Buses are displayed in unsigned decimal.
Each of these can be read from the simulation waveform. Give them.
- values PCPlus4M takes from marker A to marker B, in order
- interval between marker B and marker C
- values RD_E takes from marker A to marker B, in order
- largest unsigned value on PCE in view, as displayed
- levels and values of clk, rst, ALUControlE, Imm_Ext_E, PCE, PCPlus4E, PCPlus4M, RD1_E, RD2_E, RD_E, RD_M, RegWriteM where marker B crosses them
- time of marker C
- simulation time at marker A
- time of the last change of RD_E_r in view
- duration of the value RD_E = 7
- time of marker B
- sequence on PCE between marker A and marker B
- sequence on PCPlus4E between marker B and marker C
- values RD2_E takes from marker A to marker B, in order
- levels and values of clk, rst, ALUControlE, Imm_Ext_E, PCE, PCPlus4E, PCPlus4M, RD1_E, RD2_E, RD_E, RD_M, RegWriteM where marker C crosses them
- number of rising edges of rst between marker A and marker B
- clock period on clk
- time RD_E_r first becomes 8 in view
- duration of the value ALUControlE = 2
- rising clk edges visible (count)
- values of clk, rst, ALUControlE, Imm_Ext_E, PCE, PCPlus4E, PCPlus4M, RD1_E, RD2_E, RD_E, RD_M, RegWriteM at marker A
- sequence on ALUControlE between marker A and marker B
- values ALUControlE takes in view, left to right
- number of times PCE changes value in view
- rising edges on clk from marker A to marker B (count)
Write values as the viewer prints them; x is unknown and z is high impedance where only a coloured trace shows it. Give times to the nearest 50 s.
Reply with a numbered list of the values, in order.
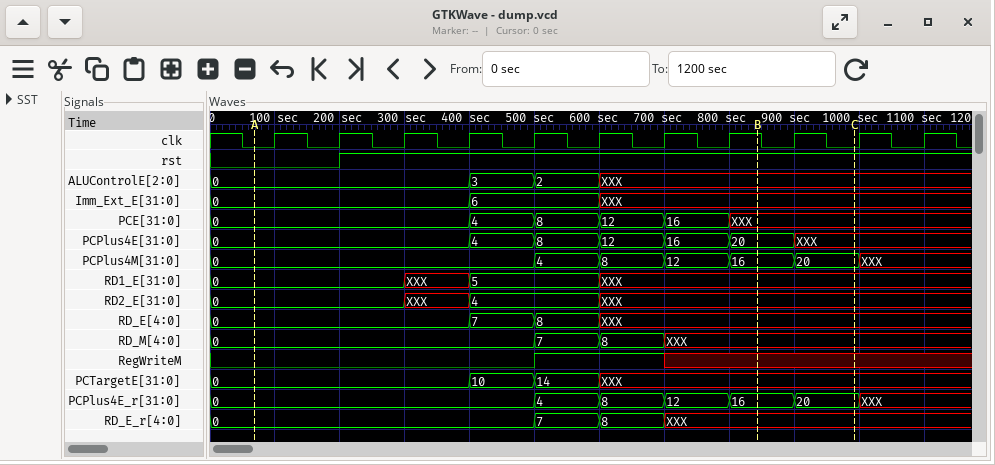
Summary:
1. 0, 4, 8, 12, 16
2. 150 s
3. 0, 7, 8, XXX
4. 16
5. clk=1, rst=1, ALUControlE=XXX, Imm_Ext_E=XXX, PCE=XXX, PCPlus4E=20, PCPlus4M=16, RD1_E=XXX, RD2_E=XXX, RD_E=XXX, RD_M=XXX, RegWriteM=x
6. 1000 s
7. 50 s
8. 700 s
9. 100 s
10. 850 s
11. 0, 4, 8, 12, 16, XXX
12. 20, XXX
13. 0, XXX, 4, XXX
14. clk=0, rst=1, ALUControlE=XXX, Imm_Ext_E=XXX, PCE=XXX, PCPlus4E=XXX, PCPlus4M=20, RD1_E=XXX, RD2_E=XXX, RD_E=XXX, RD_M=XXX, RegWriteM=x
15. 1
16. 100 s
17. 600 s
18. 100 s
19. 11
20. clk=0, rst=0, ALUControlE=0, Imm_Ext_E=0, PCE=0, PCPlus4E=0, PCPlus4M=0, RD1_E=0, RD2_E=0, RD_E=0, RD_M=0, RegWriteM=0
21. 0, 3, 2, XXX
22. 0, 3, 2, XXX
23. 5
24. 8
